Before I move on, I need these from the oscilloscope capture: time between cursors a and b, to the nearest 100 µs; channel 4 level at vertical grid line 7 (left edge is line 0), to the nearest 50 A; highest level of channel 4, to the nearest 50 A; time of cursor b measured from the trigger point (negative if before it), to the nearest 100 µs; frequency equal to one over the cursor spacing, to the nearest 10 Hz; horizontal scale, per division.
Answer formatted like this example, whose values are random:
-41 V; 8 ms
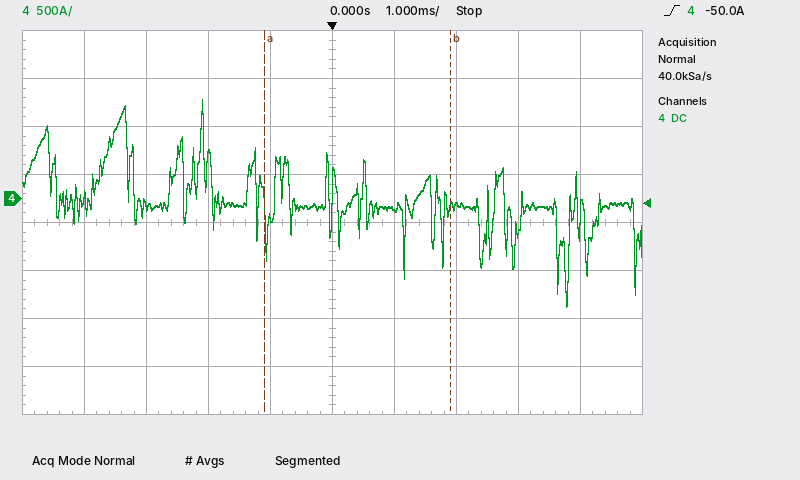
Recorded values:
3.0 ms; -100 A; 1.05 kA; +1.9 ms; 330 Hz; 1 ms
